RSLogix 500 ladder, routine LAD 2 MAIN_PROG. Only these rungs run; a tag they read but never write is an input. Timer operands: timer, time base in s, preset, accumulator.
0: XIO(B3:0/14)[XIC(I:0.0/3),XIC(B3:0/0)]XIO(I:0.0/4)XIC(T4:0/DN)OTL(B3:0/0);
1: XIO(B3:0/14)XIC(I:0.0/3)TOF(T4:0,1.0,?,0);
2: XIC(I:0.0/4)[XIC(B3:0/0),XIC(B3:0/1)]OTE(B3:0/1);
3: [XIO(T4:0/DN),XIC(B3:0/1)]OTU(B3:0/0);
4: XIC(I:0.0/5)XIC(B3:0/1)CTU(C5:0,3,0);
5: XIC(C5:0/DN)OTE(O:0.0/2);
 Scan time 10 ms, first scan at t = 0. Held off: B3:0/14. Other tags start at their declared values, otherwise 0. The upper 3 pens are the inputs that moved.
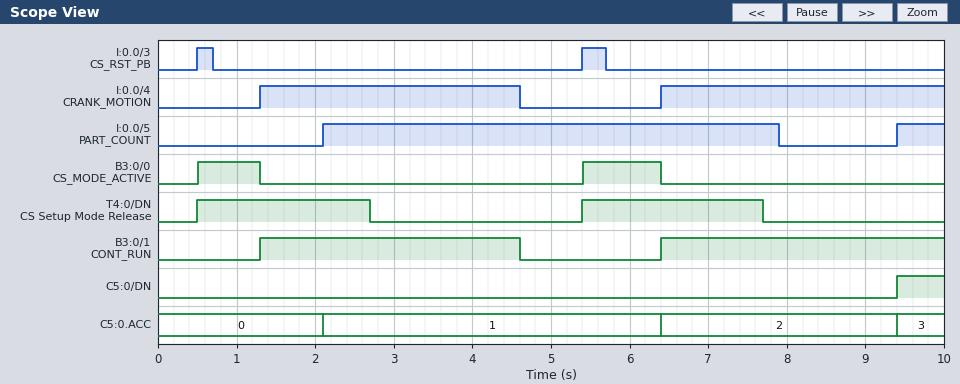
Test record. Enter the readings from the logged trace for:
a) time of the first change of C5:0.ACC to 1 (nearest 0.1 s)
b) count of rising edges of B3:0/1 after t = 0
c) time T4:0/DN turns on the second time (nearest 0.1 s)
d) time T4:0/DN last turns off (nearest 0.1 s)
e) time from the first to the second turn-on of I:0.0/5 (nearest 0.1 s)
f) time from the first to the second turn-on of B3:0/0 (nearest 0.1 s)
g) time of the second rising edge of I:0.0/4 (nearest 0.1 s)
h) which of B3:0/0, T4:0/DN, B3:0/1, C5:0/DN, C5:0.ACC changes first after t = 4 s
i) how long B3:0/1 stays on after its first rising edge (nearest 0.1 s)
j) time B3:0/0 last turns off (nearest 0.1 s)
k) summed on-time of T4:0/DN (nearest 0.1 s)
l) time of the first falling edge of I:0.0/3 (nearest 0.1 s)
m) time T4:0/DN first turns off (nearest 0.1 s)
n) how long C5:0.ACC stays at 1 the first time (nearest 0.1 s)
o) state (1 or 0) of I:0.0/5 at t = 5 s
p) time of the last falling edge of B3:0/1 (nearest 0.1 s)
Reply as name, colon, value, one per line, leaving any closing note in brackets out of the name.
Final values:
time of the first change of C5:0.ACC to 1: 2.1 s
count of rising edges of B3:0/1 after t = 0: 2
time T4:0/DN turns on the second time: 5.4 s
time T4:0/DN last turns off: 7.7 s
time from the first to the second turn-on of I:0.0/5: 7.3 s
time from the first to the second turn-on of B3:0/0: 4.9 s
time of the second rising edge of I:0.0/4: 6.4 s
which of B3:0/0, T4:0/DN, B3:0/1, C5:0/DN, C5:0.ACC changes first after t = 4 s: B3:0/1
how long B3:0/1 stays on after its first rising edge: 3.3 s
time B3:0/0 last turns off: 6.4 s
summed on-time of T4:0/DN: 4.5 s
time of the first falling edge of I:0.0/3: 0.7 s
time T4:0/DN first turns off: 2.7 s
how long C5:0.ACC stays at 1 the first time: 4.3 s
state (1 or 0) of I:0.0/5 at t = 5 s: 1
time of the last falling edge of B3:0/1: 4.6 s
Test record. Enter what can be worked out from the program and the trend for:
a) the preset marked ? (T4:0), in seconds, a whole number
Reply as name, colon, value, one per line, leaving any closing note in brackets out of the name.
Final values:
the preset marked ? (T4:0), in seconds, a whole number: 2 s
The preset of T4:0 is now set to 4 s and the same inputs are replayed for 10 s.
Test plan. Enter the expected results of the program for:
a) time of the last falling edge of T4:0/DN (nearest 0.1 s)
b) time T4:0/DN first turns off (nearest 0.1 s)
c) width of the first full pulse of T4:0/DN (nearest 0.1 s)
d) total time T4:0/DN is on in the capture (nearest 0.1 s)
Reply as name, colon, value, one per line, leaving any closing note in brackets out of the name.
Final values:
time of the last falling edge of T4:0/DN: 9.7 s
time T4:0/DN first turns off: 4.7 s
width of the first full pulse of T4:0/DN: 4.2 s
total time T4:0/DN is on in the capture: 8.5 s
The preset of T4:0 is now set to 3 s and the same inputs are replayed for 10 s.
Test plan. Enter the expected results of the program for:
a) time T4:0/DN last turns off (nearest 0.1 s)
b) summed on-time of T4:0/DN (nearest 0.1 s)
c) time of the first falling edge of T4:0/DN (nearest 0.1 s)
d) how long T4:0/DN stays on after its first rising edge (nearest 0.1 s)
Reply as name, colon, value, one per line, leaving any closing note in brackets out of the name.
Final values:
time T4:0/DN last turns off: 8.7 s
summed on-time of T4:0/DN: 6.5 s
time of the first falling edge of T4:0/DN: 3.7 s
how long T4:0/DN stays on after its first rising edge: 3.2 s
